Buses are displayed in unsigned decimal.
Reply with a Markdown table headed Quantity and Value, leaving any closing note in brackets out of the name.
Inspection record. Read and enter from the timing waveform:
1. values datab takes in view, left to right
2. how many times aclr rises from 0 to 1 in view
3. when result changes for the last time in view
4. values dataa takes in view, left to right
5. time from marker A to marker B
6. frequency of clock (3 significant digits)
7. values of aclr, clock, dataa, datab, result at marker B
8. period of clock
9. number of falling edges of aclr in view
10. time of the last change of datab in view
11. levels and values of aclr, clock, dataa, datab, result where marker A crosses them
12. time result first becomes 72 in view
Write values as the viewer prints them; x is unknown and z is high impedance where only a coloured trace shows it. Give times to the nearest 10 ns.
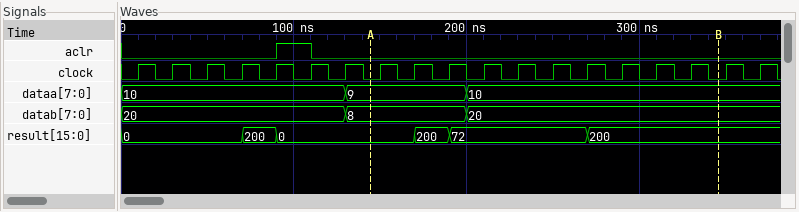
| Quantity | Value |
|---|---|
| values datab takes in view, left to right | 20, 8, 20 |
| how many times aclr rises from 0 to 1 in view | 1 |
| when result changes for the last time in view | 270 ns |
| values dataa takes in view, left to right | 10, 9, 10 |
| time from marker A to marker B | 200 ns |
| frequency of clock | 50.0 MHz |
| values of aclr, clock, dataa, datab, result at marker B | aclr=0, clock=0, dataa=10, datab=20, result=200 |
| period of clock | 20 ns |
| number of falling edges of aclr in view | 1 |
| time of the last change of datab in view | 200 ns |
| levels and values of aclr, clock, dataa, datab, result where marker A crosses them | aclr=0, clock=0, dataa=9, datab=8, result=0 |
| time result first becomes 72 in view | 190 ns |
